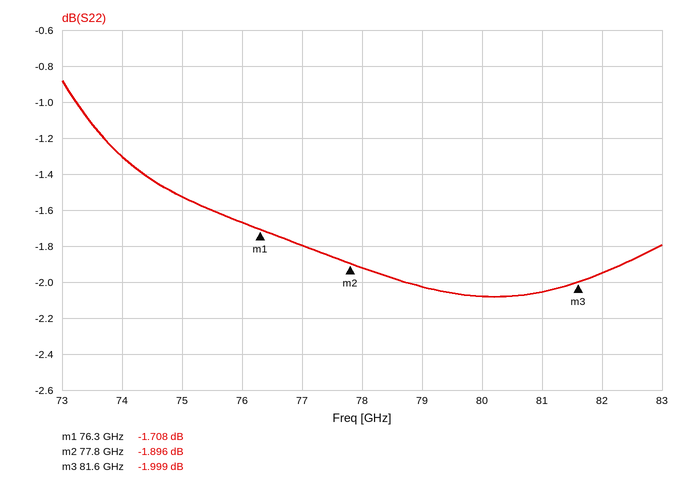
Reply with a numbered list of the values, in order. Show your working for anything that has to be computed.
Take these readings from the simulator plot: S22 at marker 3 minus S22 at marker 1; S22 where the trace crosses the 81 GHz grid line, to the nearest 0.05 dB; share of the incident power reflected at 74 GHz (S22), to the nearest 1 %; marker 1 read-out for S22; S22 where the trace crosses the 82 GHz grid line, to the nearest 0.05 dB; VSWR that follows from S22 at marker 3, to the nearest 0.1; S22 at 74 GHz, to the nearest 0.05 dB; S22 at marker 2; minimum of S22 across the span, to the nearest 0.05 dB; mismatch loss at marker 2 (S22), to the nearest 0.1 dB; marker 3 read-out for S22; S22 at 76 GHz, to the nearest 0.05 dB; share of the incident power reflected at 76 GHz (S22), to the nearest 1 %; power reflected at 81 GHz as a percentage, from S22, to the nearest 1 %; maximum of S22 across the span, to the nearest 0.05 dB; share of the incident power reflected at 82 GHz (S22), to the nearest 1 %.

1. -1.999 − (-1.708) = -0.291 dB
2. -2.05 dB
3. 10^(-1.3/10) ≈ 74 %
4. -1.708 dB
5. -1.95 dB
6. (1 + 0.7944)/(1 − 0.7944) ≈ 8.7
7. -1.30 dB
8. -1.896 dB
9. -2.10 dB
10. −10 log10(1 − 10^(-1.896/10)) ≈ 4.5 dB
11. -1.999 dB
12. -1.65 dB
13. 10^(-1.65/10) ≈ 68 %
14. 10^(-2.05/10) ≈ 62 %
15. -0.90 dB
16. 10^(-1.95/10) ≈ 64 %
